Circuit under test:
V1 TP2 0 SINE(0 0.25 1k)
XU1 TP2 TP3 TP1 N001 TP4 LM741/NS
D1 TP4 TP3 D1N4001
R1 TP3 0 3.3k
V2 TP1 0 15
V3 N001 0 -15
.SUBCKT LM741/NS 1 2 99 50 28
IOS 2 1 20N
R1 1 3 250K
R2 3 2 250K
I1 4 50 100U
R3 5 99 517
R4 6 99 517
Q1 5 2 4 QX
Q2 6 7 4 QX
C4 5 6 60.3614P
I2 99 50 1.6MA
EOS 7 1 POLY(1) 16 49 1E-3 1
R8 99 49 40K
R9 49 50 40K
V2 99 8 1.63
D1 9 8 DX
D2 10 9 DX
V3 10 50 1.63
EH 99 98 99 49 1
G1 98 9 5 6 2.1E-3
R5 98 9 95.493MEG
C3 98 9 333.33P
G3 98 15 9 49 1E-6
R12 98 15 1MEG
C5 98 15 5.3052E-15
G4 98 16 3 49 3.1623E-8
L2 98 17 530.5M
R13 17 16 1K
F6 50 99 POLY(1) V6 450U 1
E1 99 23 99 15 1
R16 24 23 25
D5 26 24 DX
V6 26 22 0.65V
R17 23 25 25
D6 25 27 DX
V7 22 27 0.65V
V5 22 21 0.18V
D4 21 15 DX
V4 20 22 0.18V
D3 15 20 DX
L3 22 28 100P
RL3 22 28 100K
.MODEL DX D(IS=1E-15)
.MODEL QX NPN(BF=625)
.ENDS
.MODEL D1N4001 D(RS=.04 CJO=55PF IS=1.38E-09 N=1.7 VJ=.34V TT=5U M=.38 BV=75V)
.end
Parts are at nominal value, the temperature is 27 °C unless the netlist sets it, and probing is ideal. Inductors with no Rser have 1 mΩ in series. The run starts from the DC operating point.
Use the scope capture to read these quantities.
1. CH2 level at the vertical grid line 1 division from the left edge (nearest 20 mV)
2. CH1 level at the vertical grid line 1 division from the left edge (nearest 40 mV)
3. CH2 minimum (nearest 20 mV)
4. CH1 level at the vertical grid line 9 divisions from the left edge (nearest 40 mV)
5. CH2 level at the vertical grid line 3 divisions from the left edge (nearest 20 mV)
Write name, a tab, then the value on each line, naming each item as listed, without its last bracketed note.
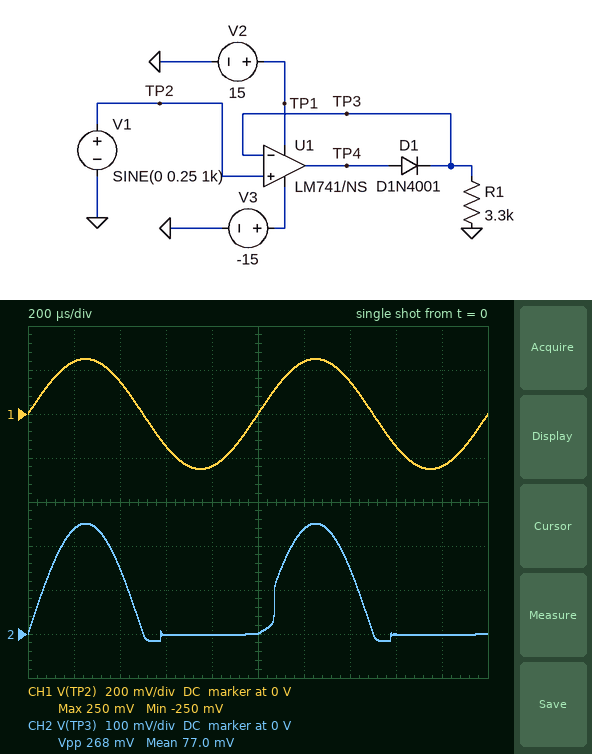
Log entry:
CH2 level at the vertical grid line 1 division from the left edge	240 mV
CH1 level at the vertical grid line 1 division from the left edge	240 mV
CH2 minimum	-20 mV
CH1 level at the vertical grid line 9 divisions from the left edge	-240 mV
CH2 level at the vertical grid line 3 divisions from the left edge	0 V
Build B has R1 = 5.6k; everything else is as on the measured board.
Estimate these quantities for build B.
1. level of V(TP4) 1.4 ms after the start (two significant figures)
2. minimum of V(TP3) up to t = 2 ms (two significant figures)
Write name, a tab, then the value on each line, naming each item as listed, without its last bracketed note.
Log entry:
level of V(TP4) 1.4 ms after the start	580 mV
minimum of V(TP3) up to t = 2 ms	-27 mV
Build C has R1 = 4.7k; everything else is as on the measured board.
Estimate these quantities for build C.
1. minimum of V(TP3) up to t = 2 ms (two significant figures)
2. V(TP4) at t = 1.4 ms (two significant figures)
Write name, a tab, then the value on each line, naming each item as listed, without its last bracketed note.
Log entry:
minimum of V(TP3) up to t = 2 ms	-23 mV
V(TP4) at t = 1.4 ms	590 mV
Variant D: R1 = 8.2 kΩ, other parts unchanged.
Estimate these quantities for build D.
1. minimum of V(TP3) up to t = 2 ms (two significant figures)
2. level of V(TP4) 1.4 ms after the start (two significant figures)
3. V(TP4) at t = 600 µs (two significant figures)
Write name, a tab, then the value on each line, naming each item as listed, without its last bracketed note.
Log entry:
minimum of V(TP3) up to t = 2 ms	-39 mV
level of V(TP4) 1.4 ms after the start	570 mV
V(TP4) at t = 600 µs	-14 V
